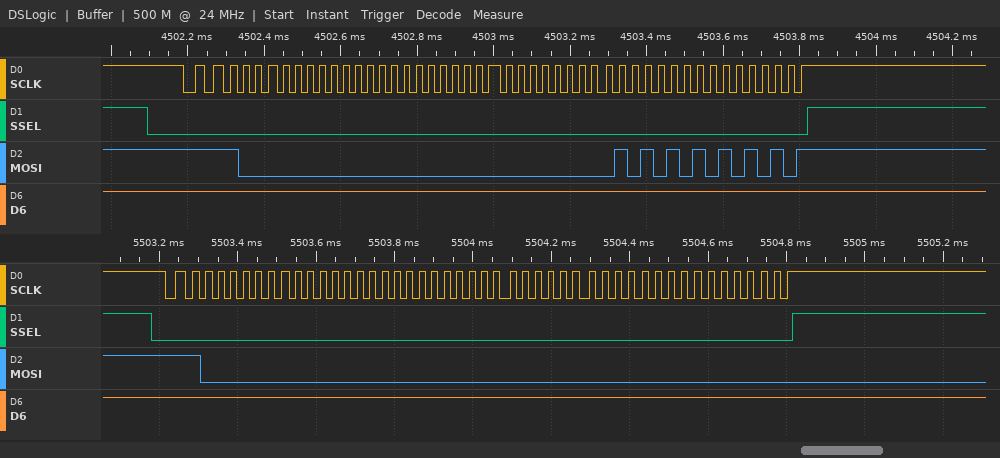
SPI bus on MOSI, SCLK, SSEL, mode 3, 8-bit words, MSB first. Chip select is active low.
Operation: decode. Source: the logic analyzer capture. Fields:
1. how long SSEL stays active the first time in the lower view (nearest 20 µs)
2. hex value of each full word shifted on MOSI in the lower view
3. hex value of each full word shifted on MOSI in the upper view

1640 µs
C0, 00, 00, 00, 00, 00
E0, 00, 00, 00, 55, 55
